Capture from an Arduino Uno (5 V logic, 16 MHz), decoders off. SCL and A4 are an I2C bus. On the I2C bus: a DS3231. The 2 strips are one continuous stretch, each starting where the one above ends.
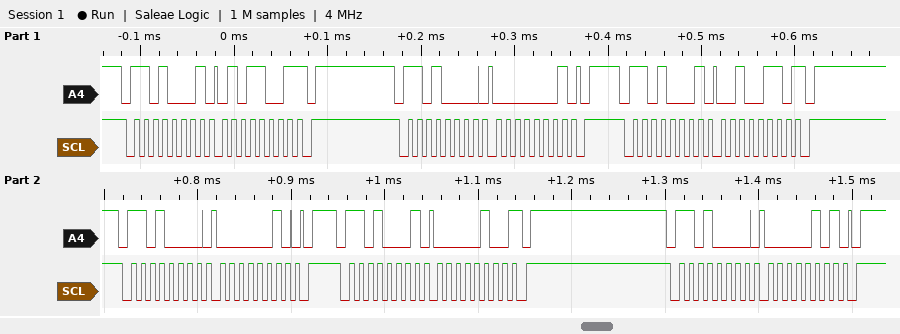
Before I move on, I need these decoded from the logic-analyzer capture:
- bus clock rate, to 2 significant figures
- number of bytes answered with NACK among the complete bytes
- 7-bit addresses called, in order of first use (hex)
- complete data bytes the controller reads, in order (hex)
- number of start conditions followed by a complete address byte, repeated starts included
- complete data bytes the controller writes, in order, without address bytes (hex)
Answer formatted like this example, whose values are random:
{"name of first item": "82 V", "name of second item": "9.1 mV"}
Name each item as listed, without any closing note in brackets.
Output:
{"bus clock rate, to 2 significant figures": "100 kHz", "number of bytes answered with NACK among the complete bytes": "3", "7-bit addresses called, in order of first use": "0x68", "complete data bytes the controller reads, in order": "59 26 04", "number of start conditions followed by a complete address byte, repeated starts included": "6", "complete data bytes the controller writes, in order, without address bytes": "01 02 05"}
